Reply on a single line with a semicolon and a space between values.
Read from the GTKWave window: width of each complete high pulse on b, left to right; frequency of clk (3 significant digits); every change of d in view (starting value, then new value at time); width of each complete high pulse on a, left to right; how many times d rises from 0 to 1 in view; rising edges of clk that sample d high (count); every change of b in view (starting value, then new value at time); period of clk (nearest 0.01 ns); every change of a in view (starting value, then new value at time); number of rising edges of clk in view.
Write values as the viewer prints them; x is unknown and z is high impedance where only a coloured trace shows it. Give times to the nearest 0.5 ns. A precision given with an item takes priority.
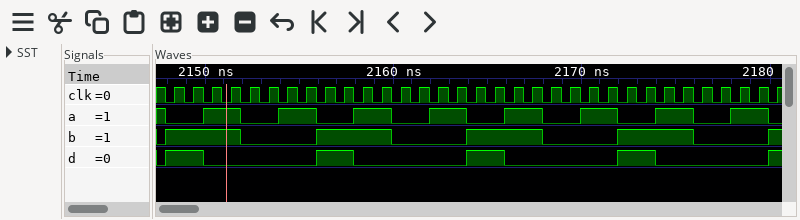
4 ns, 4 ns, 4 ns, 4 ns; 1.00 GHz; 0, 1 at 2148 ns, 0 at 2150 ns, 1 at 2156 ns, 0 at 2158 ns, 1 at 2164 ns, 0 at 2166 ns, 1 at 2172 ns, 0 at 2174 ns, 1 at 2180 ns; 2 ns, 2 ns, 2 ns, 2 ns, 2 ns, 2 ns, 2 ns, 2 ns; 5; 9; 0, 1 at 2148 ns, 0 at 2152 ns, 1 at 2156 ns, 0 at 2160 ns, 1 at 2164 ns, 0 at 2168 ns, 1 at 2172 ns, 0 at 2176 ns, 1 at 2180 ns; 1 ns; 1, 0 at 2148 ns, 1 at 2150 ns, 0 at 2152 ns, 1 at 2154 ns, 0 at 2156 ns, 1 at 2158 ns, 0 at 2160 ns, 1 at 2162 ns, 0 at 2164 ns, 1 at 2166 ns, 0 at 2168 ns, 1 at 2170 ns, 0 at 2172 ns, 1 at 2174 ns, 0 at 2176 ns, 1 at 2178 ns, 0 at 2180 ns; 33
